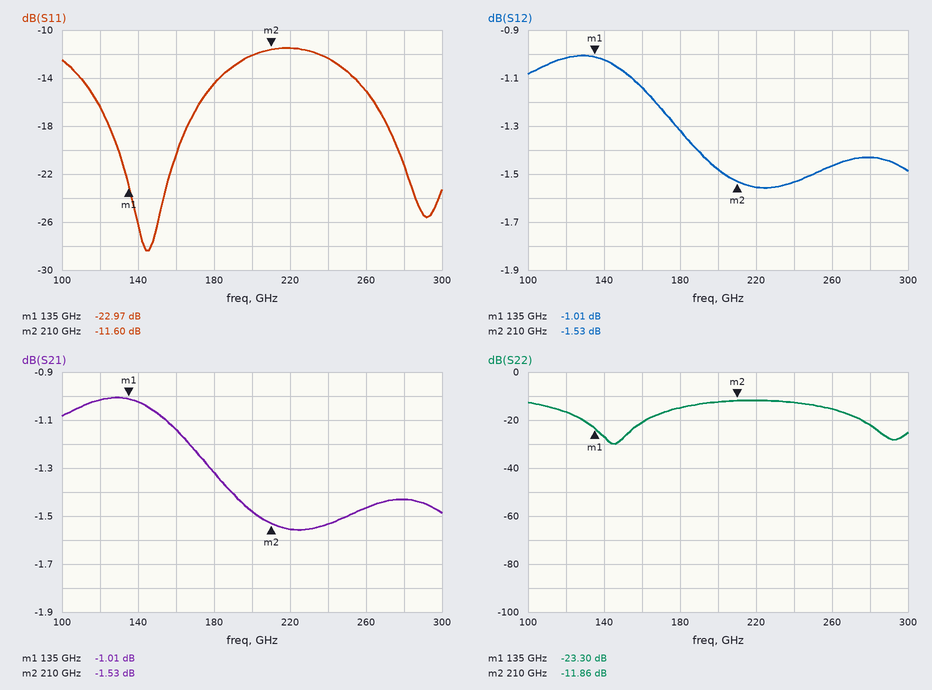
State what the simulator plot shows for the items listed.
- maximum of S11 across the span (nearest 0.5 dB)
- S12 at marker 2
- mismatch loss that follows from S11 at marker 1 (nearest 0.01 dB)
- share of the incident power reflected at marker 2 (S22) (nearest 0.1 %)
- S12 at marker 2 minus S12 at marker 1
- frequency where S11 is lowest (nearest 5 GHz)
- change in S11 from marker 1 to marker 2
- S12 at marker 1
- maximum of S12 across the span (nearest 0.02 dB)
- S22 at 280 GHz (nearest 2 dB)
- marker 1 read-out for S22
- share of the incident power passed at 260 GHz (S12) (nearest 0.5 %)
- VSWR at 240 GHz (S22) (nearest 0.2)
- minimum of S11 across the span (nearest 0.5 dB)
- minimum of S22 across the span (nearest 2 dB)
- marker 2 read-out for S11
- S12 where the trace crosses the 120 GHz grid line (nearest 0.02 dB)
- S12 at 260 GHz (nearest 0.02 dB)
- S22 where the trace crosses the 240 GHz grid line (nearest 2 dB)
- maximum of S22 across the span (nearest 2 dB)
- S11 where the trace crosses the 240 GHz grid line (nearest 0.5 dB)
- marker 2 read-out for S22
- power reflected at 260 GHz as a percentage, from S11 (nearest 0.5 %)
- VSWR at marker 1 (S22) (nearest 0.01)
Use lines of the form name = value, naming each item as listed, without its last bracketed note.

maximum of S11 across the span = -11.5 dB
S12 at marker 2 = -1.53 dB
mismatch loss that follows from S11 at marker 1 = 0.02 dB
share of the incident power reflected at marker 2 (S22) = 6.5 %
S12 at marker 2 minus S12 at marker 1 = -0.52 dB
frequency where S11 is lowest = 145 GHz
change in S11 from marker 1 to marker 2 = 11.37 dB
S12 at marker 1 = -1.01 dB
maximum of S12 across the span = -1.00 dB
S22 at 280 GHz = -22 dB
marker 1 read-out for S22 = -23.30 dB
share of the incident power passed at 260 GHz (S12) = 71.5 %
VSWR at 240 GHz (S22) = 1.6
minimum of S11 across the span = -28.5 dB
minimum of S22 across the span = -30 dB
marker 2 read-out for S11 = -11.60 dB
S12 where the trace crosses the 120 GHz grid line = -1.02 dB
S12 at 260 GHz = -1.46 dB
S22 where the trace crosses the 240 GHz grid line = -12 dB
maximum of S22 across the span = -12 dB
S11 where the trace crosses the 240 GHz grid line = -12.5 dB
marker 2 read-out for S22 = -11.86 dB
power reflected at 260 GHz as a percentage, from S11 = 3.0 %
VSWR at marker 1 (S22) = 1.15
